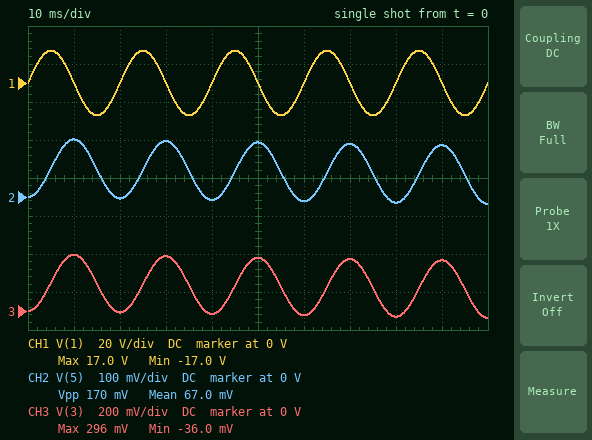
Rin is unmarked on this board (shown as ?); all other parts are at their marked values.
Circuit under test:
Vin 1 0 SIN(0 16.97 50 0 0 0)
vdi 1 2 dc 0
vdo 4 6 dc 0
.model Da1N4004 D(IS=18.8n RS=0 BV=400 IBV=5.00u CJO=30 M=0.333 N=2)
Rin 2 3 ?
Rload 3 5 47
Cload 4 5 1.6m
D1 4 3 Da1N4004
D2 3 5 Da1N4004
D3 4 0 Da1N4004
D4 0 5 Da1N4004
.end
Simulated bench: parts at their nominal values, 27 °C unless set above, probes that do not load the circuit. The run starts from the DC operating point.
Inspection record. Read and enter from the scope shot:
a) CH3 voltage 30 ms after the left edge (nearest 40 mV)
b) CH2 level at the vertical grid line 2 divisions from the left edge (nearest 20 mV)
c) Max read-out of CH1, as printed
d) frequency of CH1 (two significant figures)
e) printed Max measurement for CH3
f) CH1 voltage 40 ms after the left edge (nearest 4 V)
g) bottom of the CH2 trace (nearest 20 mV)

280 mV
0 V
17.0 V
50 Hz
296 mV
0 V
-20 mV
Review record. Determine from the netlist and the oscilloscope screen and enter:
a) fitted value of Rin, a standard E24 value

0.012 Ω
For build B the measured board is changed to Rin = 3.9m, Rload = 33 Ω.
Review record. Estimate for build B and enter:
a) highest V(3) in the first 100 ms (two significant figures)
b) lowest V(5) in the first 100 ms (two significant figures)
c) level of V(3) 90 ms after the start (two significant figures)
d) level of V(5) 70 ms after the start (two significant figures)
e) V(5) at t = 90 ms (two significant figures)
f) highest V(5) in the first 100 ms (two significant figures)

880 mV
-130 mV
670 mV
380 mV
360 mV
470 mV
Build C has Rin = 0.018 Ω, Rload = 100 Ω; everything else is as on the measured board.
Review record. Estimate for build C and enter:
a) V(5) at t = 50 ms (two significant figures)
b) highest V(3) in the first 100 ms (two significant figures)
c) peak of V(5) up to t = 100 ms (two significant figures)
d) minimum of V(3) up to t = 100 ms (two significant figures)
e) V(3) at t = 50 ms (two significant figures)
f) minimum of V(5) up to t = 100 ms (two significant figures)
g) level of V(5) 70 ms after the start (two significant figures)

97 mV
200 mV
100 mV
-17 mV
190 mV
-8.4 mV
95 mV
